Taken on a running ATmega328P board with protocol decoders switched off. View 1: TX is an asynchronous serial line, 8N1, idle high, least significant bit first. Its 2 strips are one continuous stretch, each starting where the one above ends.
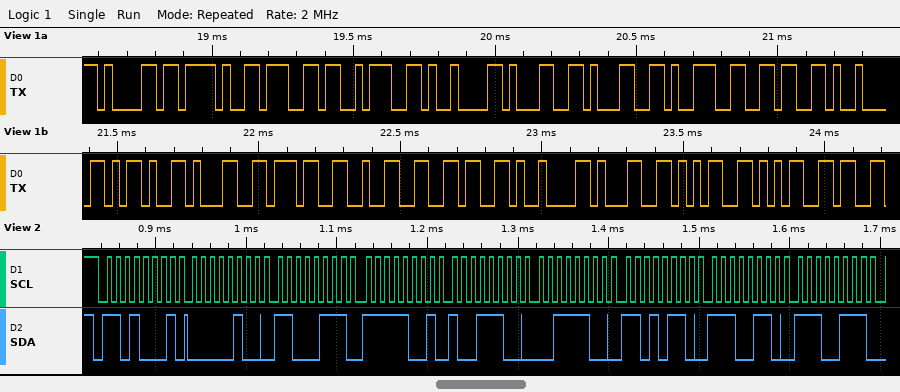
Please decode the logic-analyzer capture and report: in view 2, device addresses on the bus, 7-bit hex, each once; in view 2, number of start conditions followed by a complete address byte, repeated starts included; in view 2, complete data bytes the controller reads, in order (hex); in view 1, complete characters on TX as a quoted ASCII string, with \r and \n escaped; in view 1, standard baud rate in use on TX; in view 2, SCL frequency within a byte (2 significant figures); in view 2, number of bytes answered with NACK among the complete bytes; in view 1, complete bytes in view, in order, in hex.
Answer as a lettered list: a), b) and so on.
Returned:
a) 0x68
b) 1
c) 04 C7 F9 9C 3C D6 E6 E7
d) "a/g:\t1196\t-1726\t155"
e) 38400 baud
f) 100 kHz
g) 0
h) 0x61 0x2F 0x67 0x3A 0x09 0x31 0x31 0x39 0x36 0x09 0x2D 0x31 0x37 0x32 0x36 0x09 0x31 0x35 0x35
